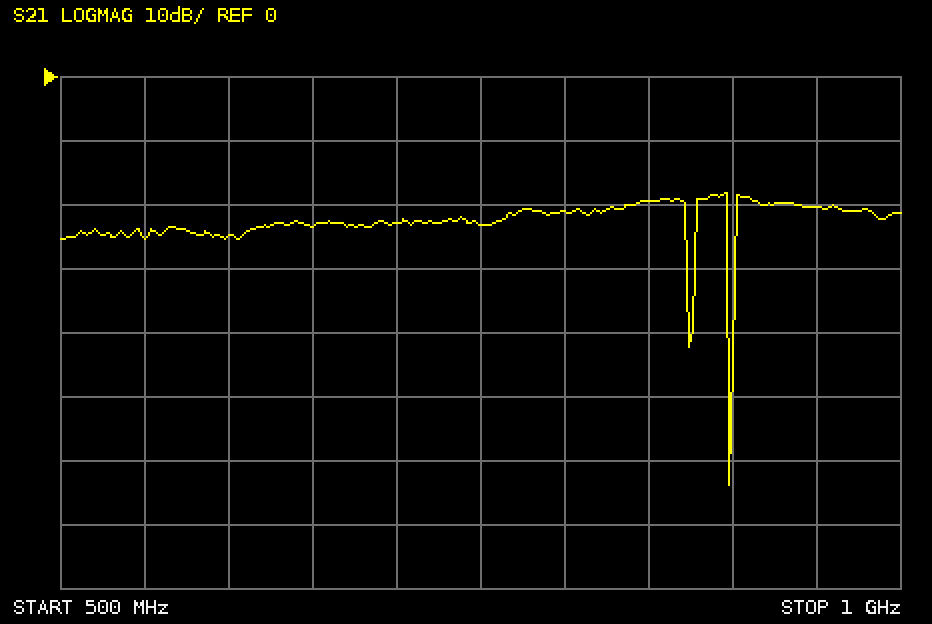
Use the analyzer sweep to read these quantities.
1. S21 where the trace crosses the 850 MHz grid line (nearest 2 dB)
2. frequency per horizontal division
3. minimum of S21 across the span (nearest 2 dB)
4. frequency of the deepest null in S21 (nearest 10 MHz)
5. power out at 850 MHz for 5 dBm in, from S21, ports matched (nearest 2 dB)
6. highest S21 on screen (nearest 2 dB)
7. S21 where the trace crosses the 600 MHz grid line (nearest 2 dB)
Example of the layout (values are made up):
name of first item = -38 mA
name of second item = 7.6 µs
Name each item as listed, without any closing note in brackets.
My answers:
S21 where the trace crosses the 850 MHz grid line = -20 dB
frequency per horizontal division = 50 MHz
minimum of S21 across the span = -64 dB
frequency of the deepest null in S21 = 900 MHz
power out at 850 MHz for 5 dBm in, from S21, ports matched = -14 dBm
highest S21 on screen = -18 dB
S21 where the trace crosses the 600 MHz grid line = -24 dB
